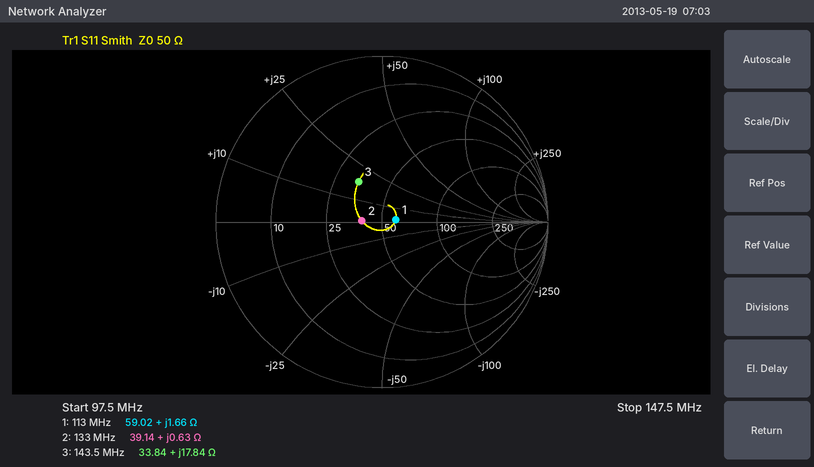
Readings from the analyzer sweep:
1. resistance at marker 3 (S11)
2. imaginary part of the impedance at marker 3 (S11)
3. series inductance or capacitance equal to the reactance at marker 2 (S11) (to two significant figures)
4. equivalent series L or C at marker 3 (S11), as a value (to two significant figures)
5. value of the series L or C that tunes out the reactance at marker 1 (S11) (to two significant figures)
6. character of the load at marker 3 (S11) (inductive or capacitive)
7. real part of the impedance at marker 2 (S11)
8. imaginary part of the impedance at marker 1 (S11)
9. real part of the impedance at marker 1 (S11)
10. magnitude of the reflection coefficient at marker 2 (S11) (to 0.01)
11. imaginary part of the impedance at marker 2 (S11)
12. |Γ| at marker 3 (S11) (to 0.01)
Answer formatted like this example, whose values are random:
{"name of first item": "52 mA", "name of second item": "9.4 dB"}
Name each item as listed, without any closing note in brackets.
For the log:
{"resistance at marker 3": "33.84 Ω", "imaginary part of the impedance at marker 3": "+17.84 Ω", "series inductance or capacitance equal to the reactance at marker 2 (S11)": "750 pH", "equivalent series L or C at marker 3 (S11), as a value": "20 nH", "value of the series L or C that tunes out the reactance at marker 1 (S11)": "850 pF", "character of the load at marker 3 (S11)": "inductive", "real part of the impedance at marker 2": "39.14 Ω", "imaginary part of the impedance at marker 1": "+1.66 Ω", "real part of the impedance at marker 1": "59.02 Ω", "magnitude of the reflection coefficient at marker 2 (S11)": "0.12", "imaginary part of the impedance at marker 2": "+0.63 Ω", "|Γ| at marker 3 (S11)": "0.28"}
